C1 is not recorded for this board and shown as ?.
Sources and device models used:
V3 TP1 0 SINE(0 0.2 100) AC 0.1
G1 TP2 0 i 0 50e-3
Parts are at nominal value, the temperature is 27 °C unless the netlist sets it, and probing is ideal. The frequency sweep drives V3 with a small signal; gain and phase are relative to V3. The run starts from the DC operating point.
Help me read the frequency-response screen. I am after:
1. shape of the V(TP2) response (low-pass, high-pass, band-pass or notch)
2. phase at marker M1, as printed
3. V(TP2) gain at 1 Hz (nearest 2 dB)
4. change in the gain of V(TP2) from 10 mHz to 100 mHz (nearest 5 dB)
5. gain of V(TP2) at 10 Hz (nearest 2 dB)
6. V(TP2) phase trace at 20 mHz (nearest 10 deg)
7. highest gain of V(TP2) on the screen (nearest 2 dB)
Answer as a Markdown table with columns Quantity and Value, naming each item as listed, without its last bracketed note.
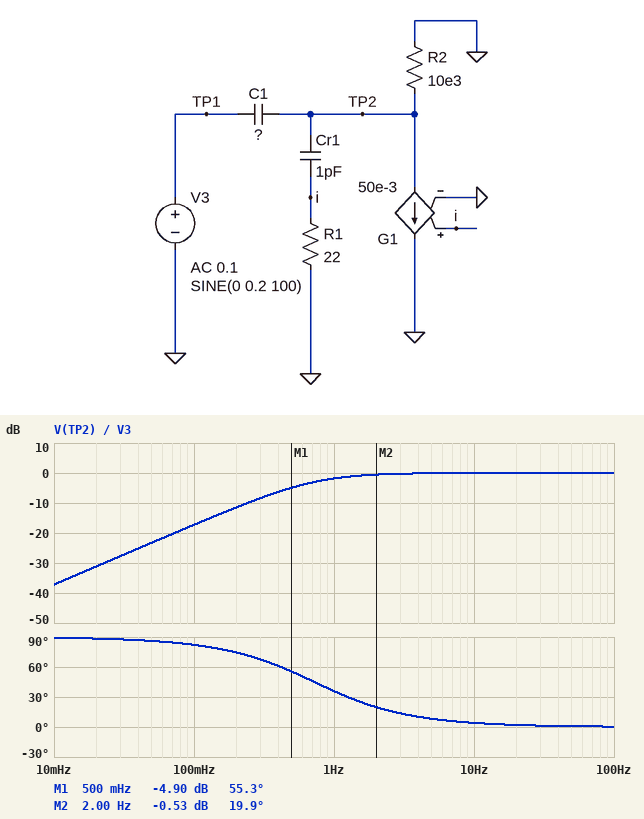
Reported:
| Quantity | Value |
|---|---|
| shape of the V(TP2) response | high-pass |
| phase at marker M1, as printed | 55.3 deg |
| V(TP2) gain at 1 Hz | -2 dB |
| change in the gain of V(TP2) from 10 mHz to 100 mHz | 20 dB |
| gain of V(TP2) at 10 Hz | 0 dB |
| V(TP2) phase trace at 20 mHz | 90 deg |
| highest gain of V(TP2) on the screen | 0 dB |
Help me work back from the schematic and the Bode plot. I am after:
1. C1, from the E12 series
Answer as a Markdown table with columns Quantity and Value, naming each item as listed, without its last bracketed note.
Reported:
| Quantity | Value |
|---|---|
| C1, from the E12 series | 22 µF |
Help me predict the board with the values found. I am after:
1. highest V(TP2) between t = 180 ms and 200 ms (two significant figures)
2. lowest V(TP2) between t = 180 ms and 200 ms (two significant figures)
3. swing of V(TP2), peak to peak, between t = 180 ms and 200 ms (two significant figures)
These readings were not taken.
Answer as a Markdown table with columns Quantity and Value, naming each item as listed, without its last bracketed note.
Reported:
| Quantity | Value |
|---|---|
| highest V(TP2) between t = 180 ms and 200 ms | 200 mV |
| lowest V(TP2) between t = 180 ms and 200 ms | -200 mV |
| swing of V(TP2), peak to peak, between t = 180 ms and 200 ms | 400 mV |
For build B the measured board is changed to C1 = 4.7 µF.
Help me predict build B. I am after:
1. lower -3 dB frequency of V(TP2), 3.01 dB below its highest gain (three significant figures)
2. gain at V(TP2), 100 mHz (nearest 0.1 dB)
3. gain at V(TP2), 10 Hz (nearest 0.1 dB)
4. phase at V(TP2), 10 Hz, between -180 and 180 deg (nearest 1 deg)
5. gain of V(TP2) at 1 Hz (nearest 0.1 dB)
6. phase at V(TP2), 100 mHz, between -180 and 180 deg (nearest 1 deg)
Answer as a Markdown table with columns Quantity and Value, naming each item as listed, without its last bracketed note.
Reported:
| Quantity | Value |
|---|---|
| lower -3 dB frequency of V(TP2), 3.01 dB below its highest gain | 3.39 Hz |
| gain at V(TP2), 100 mHz | -30.6 dB |
| gain at V(TP2), 10 Hz | -0.5 dB |
| phase at V(TP2), 10 Hz, between -180 and 180 deg | 19 deg |
| gain of V(TP2) at 1 Hz | -11.0 dB |
| phase at V(TP2), 100 mHz, between -180 and 180 deg | 88 deg |
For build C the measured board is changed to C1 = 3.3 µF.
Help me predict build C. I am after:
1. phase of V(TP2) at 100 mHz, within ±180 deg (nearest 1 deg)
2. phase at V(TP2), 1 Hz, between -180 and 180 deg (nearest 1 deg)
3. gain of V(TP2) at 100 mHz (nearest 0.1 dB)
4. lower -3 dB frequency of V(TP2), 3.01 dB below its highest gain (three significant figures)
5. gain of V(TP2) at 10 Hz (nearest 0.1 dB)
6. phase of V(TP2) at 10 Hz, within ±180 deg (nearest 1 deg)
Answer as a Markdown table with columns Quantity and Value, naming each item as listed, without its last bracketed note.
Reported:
| Quantity | Value |
|---|---|
| phase of V(TP2) at 100 mHz, within ±180 deg | 89 deg |
| phase at V(TP2), 1 Hz, between -180 and 180 deg | 78 deg |
| gain of V(TP2) at 100 mHz | -33.7 dB |
| lower -3 dB frequency of V(TP2), 3.01 dB below its highest gain | 4.82 Hz |
| gain of V(TP2) at 10 Hz | -0.9 dB |
| phase of V(TP2) at 10 Hz, within ±180 deg | 26 deg |
